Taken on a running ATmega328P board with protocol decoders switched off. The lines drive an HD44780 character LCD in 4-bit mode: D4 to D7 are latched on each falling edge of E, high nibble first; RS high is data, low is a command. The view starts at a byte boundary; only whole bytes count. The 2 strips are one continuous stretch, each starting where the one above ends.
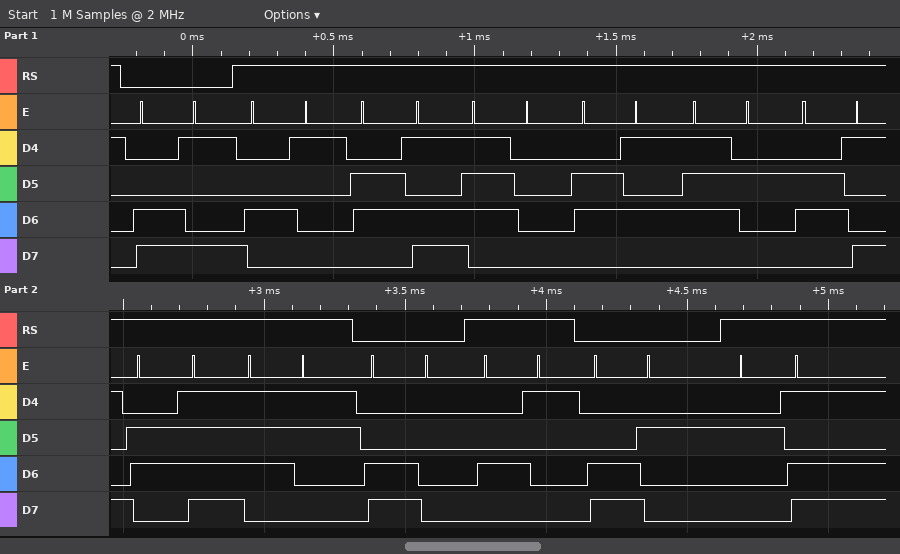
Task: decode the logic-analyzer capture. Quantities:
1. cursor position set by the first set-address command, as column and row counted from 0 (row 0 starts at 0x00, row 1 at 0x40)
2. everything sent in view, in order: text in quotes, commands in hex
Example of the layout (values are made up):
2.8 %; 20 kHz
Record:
column 9, row 1; 0xC9 "Amperios" 0xC0 "A" 0xC2 "-"
